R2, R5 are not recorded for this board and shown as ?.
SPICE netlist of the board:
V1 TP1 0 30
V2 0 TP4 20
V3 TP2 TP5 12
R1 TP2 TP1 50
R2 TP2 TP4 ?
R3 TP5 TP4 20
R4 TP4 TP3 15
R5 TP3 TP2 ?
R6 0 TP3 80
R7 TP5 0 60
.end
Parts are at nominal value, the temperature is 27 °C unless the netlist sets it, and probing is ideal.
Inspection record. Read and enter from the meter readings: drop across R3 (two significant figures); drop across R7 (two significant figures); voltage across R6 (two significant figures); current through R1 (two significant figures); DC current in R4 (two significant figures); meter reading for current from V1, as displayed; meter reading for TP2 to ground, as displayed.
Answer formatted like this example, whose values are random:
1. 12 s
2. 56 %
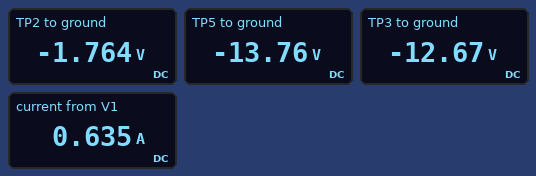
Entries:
1. 6.2 V
2. 14 V
3. 13 V
4. 640 mA
5. 490 mA
6. 0.635 A
7. -1.764 V
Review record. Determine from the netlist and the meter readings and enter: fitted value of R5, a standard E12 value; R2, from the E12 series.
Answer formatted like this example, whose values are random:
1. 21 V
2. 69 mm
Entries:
1. 33 Ω
2. 82 Ω
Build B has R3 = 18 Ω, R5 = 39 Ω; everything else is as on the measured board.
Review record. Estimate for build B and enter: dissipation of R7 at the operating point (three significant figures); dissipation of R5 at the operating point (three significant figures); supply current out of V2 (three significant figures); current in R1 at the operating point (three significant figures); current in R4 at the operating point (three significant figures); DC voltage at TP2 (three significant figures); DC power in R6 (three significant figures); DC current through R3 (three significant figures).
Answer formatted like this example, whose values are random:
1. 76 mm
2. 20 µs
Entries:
1. 3.14 W
2. 3.34 W
3. 1.03 A
4. 635 mA
5. 457 mA
6. -1.73 V
7. 2.16 W
8. 348 mA
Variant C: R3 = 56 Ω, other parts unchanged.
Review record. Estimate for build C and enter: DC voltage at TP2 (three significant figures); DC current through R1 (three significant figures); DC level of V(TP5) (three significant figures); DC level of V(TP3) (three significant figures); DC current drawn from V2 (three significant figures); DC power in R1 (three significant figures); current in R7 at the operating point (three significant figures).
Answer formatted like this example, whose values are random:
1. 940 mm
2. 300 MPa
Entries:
1. 498 mV
2. 590 mA
3. -11.5 V
4. -12.0 V
5. 932 mA
6. 17.4 W
7. 192 mA
